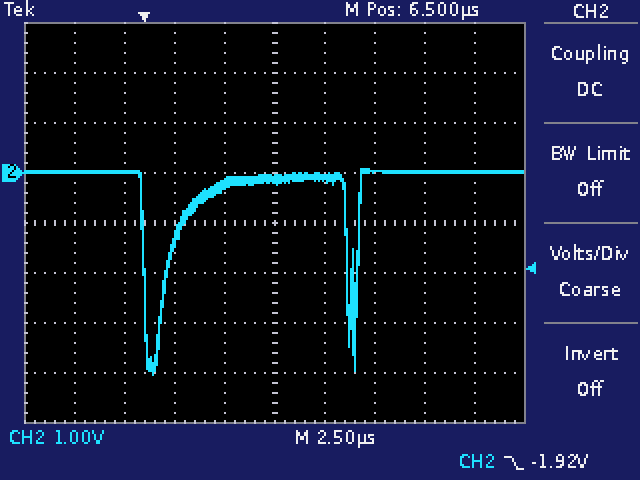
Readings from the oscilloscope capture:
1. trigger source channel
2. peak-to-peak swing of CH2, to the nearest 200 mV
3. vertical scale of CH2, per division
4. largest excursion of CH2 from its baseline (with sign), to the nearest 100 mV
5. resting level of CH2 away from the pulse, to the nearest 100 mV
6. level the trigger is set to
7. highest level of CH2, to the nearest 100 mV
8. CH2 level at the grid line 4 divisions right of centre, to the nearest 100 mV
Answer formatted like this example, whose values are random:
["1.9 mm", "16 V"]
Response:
["CH2", "4.2 V", "1 V", "-4.1 V", "0.0 V", "-1.92 V", "100 mV", "0.0 V"]
